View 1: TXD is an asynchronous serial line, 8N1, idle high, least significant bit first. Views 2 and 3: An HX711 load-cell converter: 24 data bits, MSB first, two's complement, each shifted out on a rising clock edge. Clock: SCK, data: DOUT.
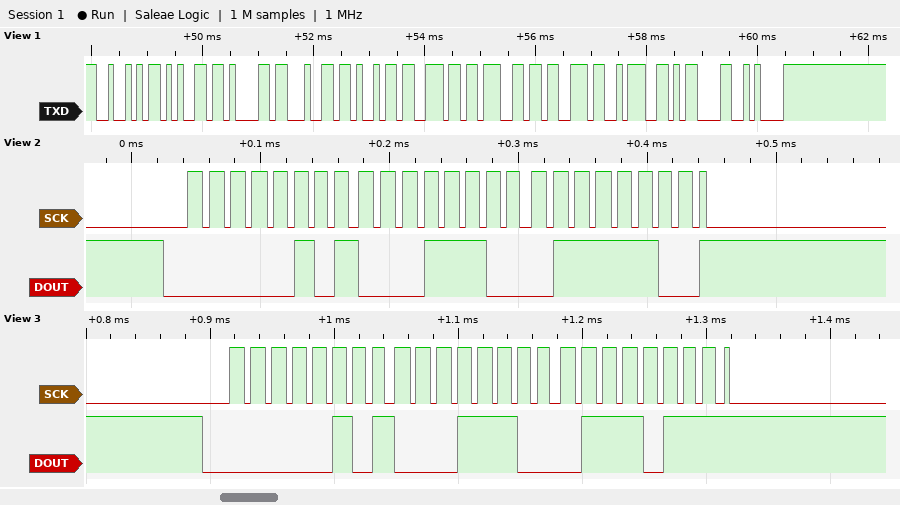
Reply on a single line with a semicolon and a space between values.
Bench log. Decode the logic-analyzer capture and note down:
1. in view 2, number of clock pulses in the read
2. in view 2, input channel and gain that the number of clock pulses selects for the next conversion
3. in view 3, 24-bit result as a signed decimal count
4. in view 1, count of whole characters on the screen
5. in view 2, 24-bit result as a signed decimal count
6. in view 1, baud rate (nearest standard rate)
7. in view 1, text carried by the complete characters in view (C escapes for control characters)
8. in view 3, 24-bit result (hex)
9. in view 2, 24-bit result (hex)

25; channel A, gain 128; 334967; 11; 334972; 9600 baud; "Readings:\r\n"; 0x051C77; 0x051C7C
